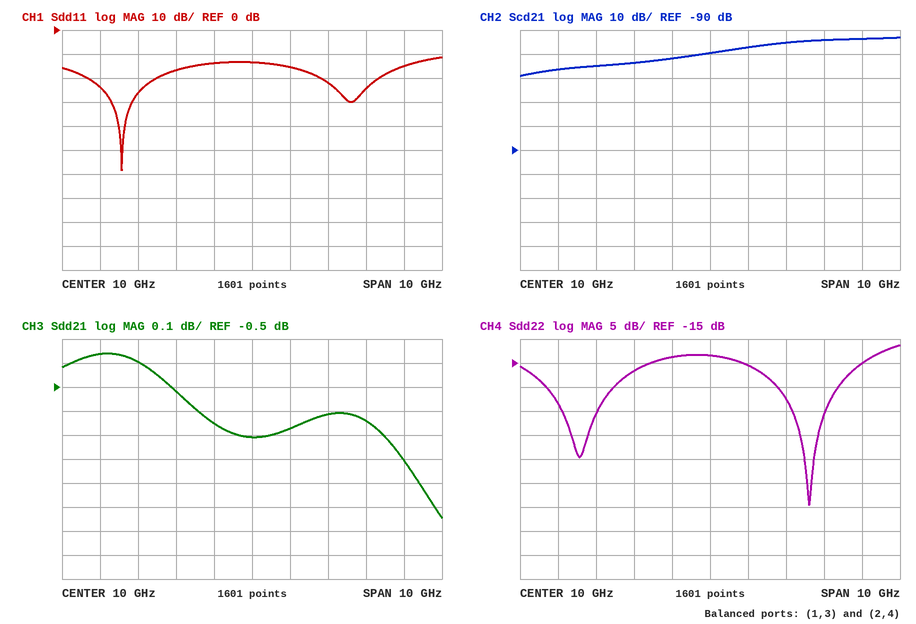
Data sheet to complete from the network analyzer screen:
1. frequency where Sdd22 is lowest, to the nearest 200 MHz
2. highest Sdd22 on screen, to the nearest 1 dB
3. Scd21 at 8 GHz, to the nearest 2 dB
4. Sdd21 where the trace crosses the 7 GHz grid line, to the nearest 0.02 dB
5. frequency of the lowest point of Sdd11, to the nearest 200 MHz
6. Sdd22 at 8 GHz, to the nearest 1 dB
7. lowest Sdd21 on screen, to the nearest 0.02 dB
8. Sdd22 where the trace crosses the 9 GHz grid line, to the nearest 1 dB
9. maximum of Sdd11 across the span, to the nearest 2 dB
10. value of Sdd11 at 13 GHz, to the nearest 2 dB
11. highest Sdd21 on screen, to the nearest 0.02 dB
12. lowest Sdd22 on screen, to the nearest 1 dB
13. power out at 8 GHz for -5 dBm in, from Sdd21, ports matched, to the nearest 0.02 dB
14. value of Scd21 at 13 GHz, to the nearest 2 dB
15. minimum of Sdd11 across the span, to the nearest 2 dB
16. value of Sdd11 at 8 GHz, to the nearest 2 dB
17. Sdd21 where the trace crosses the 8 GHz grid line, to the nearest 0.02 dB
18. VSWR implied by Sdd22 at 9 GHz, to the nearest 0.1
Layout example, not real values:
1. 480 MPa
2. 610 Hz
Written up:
1. 12.6 GHz
2. -11 dB
3. -54 dB
4. -0.40 dB
5. 6.6 GHz
6. -17 dB
7. -1.04 dB
8. -14 dB
9. -12 dB
10. -24 dB
11. -0.36 dB
12. -45 dB
13. -5.52 dBm
14. -44 dB
15. -58 dB
16. -16 dB
17. -0.52 dB
18. 1.5
